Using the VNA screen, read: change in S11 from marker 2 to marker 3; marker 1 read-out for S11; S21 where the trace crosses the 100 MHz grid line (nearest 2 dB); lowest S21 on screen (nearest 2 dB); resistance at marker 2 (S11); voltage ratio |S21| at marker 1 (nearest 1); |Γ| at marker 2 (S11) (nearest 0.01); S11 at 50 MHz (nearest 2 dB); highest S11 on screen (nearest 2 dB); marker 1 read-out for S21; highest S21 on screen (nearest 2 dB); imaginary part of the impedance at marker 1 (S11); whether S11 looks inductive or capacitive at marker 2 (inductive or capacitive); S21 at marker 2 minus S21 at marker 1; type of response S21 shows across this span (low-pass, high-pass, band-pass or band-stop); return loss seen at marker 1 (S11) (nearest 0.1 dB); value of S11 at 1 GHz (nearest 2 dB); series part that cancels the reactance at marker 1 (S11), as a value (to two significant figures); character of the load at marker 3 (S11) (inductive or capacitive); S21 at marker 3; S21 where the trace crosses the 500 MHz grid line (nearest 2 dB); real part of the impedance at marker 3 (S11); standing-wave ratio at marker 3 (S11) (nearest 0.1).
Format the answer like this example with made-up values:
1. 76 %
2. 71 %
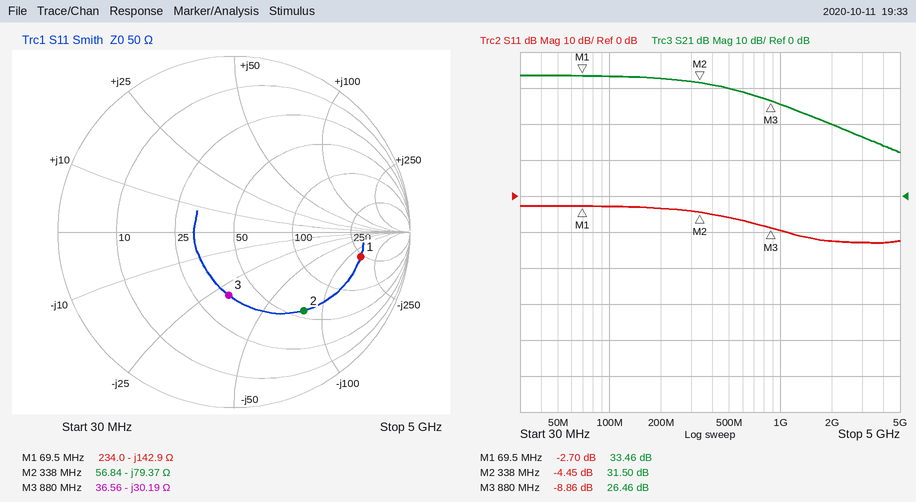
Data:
1. -4.41 dB
2. -2.70 dB
3. 34 dB
4. 12 dB
5. 56.84 Ω
6. 47
7. 0.60
8. -2 dB
9. -2 dB
10. 33.46 dB
11. 34 dB
12. -142.9 Ω
13. capacitive
14. -1.96 dB
15. low-pass
16. 2.7 dB
17. -10 dB
18. 330 nH
19. capacitive
20. 26.46 dB
21. 30 dB
22. 36.56 Ω
23. 2.1
